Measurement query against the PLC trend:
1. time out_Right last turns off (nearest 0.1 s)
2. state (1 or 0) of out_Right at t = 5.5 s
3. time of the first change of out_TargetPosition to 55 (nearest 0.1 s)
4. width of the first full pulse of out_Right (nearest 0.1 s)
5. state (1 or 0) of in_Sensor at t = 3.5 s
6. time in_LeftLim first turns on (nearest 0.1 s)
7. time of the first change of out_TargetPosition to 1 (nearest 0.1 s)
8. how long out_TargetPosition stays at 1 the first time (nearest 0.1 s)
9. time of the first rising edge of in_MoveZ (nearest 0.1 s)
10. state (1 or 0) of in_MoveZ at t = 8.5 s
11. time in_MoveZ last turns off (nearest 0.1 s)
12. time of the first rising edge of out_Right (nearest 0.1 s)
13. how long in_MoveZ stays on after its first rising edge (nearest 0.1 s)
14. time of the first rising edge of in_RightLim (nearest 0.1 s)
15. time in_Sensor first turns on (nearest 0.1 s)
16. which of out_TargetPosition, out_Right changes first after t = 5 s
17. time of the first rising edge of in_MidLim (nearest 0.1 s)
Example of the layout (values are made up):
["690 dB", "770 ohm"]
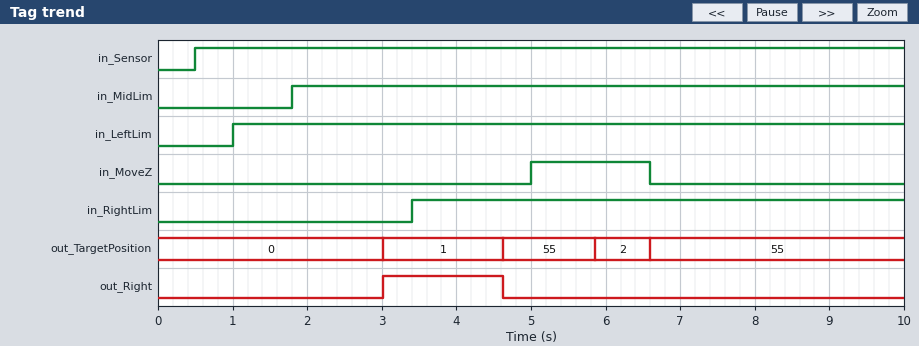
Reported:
["4.6 s", "0", "4.6 s", "1.6 s", "1", "1.0 s", "3.0 s", "1.6 s", "5.0 s", "0", "6.6 s", "3.0 s", "1.6 s", "3.4 s", "0.5 s", "out_TargetPosition", "1.8 s"]
